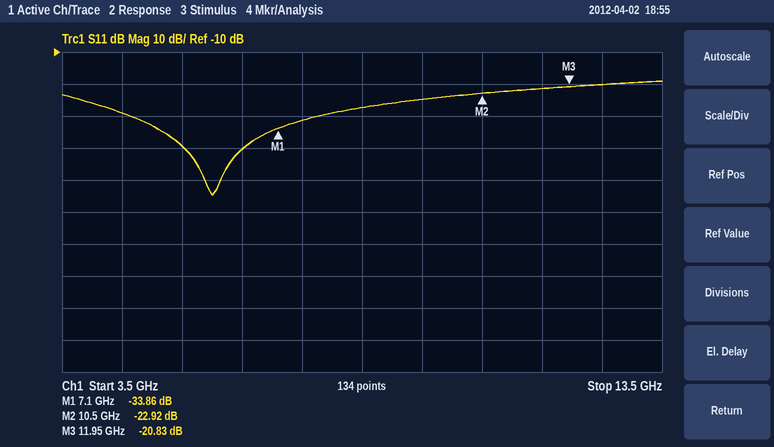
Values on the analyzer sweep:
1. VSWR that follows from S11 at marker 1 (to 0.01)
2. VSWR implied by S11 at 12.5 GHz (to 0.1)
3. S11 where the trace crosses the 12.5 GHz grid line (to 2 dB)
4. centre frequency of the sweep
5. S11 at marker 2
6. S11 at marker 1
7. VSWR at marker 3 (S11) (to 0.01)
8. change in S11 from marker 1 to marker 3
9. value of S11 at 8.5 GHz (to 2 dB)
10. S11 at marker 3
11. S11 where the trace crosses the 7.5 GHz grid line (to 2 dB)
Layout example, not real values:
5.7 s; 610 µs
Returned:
1.04; 1.2; -20 dB; 8.5 GHz; -22.92 dB; -33.86 dB; 1.20; 13.03 dB; -28 dB; -20.83 dB; -32 dB
